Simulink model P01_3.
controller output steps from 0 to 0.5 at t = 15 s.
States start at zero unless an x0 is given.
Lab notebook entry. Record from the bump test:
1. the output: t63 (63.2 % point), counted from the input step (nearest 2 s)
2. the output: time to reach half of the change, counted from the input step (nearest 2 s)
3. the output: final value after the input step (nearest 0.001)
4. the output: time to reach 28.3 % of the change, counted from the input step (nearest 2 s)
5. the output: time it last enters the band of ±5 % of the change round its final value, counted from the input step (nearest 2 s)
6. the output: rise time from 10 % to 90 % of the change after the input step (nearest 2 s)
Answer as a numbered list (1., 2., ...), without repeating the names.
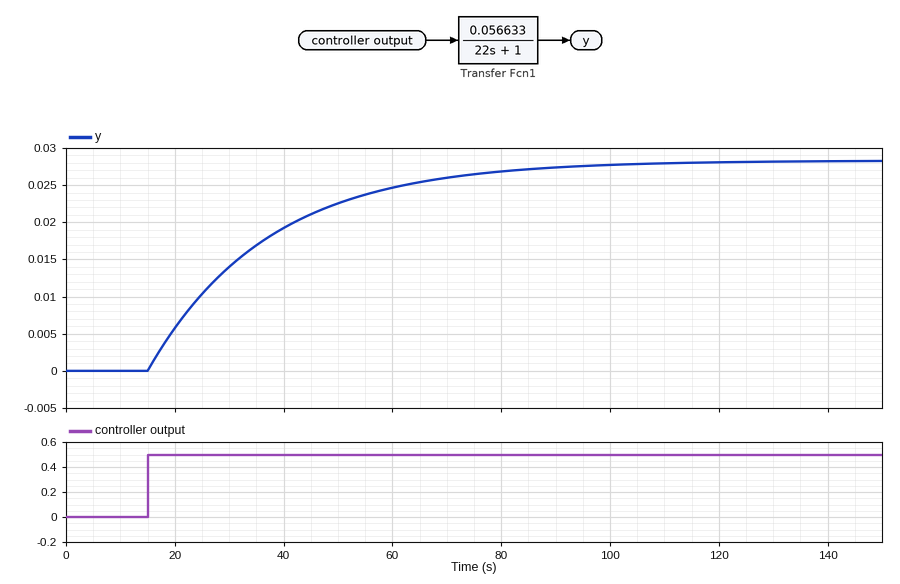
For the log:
1. 22 s
2. 16 s
3. 0.028
4. 8 s
5. 66 s
6. 48 s
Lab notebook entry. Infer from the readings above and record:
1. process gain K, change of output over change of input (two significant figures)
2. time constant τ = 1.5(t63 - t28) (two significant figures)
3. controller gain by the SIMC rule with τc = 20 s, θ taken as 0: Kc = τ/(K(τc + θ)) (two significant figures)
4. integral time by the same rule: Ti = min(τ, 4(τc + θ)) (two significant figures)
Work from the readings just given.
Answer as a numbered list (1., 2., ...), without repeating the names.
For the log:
1. 0.056
2. 21 s
3. 19
4. 21 s
